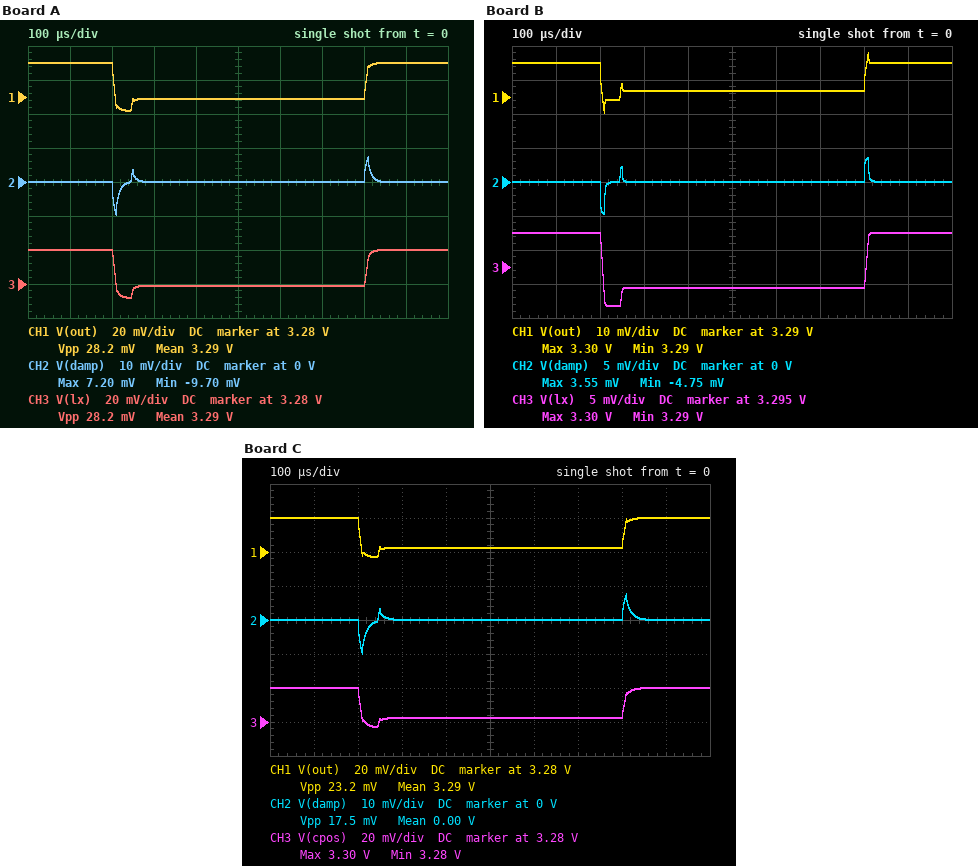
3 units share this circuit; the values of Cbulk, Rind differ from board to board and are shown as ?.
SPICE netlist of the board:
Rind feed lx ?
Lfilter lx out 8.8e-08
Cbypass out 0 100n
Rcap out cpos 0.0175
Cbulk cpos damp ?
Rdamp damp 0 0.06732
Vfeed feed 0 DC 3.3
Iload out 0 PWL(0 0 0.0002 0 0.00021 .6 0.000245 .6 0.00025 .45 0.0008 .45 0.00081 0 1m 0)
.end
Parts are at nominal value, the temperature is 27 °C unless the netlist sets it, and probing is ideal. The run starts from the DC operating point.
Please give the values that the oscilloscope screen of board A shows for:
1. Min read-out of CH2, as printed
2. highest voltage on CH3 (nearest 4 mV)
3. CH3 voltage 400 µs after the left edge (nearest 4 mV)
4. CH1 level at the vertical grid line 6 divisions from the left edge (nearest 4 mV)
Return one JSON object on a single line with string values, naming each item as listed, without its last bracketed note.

{"Min read-out of CH2, as printed": "-9.70 mV", "highest voltage on CH3": "3.300 V", "CH3 voltage 400 µs after the left edge": "3.280 V", "CH1 level at the vertical grid line 6 divisions from the left edge": "3.280 V"}
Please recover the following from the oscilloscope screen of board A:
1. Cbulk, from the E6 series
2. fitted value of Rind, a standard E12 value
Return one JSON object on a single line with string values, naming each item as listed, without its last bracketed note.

{"Cbulk, from the E6 series": "68 µF", "fitted value of Rind, a standard E12 value": "0.047 Ω"}
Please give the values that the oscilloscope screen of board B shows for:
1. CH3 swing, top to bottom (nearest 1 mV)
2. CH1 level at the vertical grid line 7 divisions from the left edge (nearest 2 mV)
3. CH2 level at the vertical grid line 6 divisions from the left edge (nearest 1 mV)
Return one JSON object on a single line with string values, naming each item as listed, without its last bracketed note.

{"CH3 swing, top to bottom": "11 mV", "CH1 level at the vertical grid line 7 divisions from the left edge": "3.292 V", "CH2 level at the vertical grid line 6 divisions from the left edge": "0 V"}
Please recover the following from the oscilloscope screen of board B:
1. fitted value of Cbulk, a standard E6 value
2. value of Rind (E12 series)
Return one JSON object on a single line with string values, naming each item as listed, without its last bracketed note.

{"fitted value of Cbulk, a standard E6 value": "68 µF", "value of Rind": "0.018 Ω"}
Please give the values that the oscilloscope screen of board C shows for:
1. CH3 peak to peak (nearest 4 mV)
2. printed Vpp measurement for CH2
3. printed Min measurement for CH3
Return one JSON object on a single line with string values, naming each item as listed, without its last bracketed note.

{"CH3 peak to peak": "24 mV", "printed Vpp measurement for CH2": "17.5 mV", "printed Min measurement for CH3": "3.28 V"}
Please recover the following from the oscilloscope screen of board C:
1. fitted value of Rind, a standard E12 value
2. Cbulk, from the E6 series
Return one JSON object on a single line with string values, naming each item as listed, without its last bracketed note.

{"fitted value of Rind, a standard E12 value": "0.039 Ω", "Cbulk, from the E6 series": "100 µF"}
